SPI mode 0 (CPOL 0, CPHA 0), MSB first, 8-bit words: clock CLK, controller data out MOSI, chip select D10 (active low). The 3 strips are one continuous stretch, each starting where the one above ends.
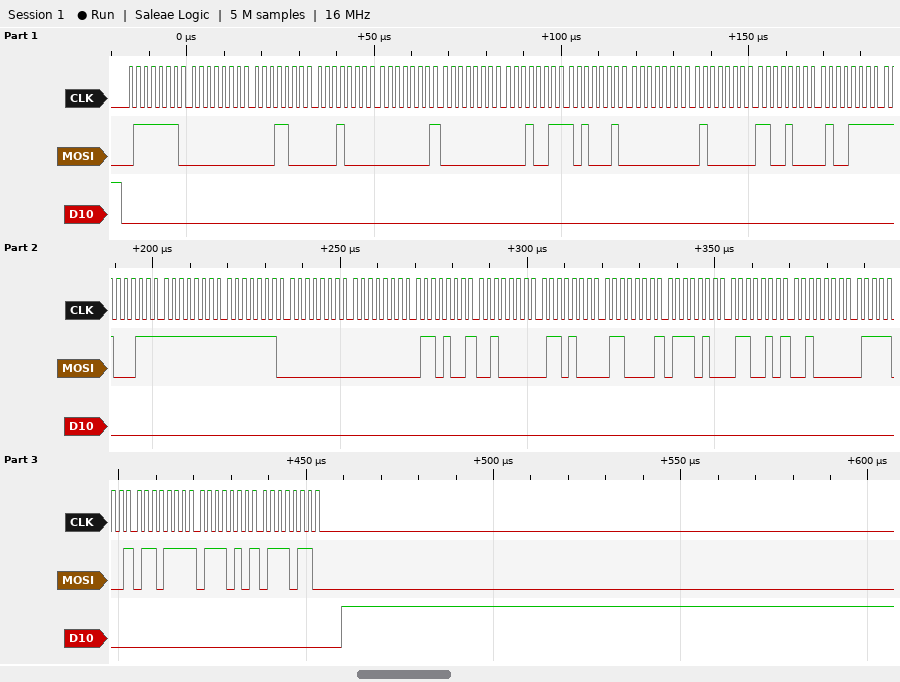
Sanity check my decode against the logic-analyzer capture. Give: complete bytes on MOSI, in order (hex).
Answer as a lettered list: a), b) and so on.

a) 7E 00 18 10 01 00 13 A2 00 40 C8 4F C7 FF FE 00 00 69 20 68 61 74 65 20 79 6F 75 76
